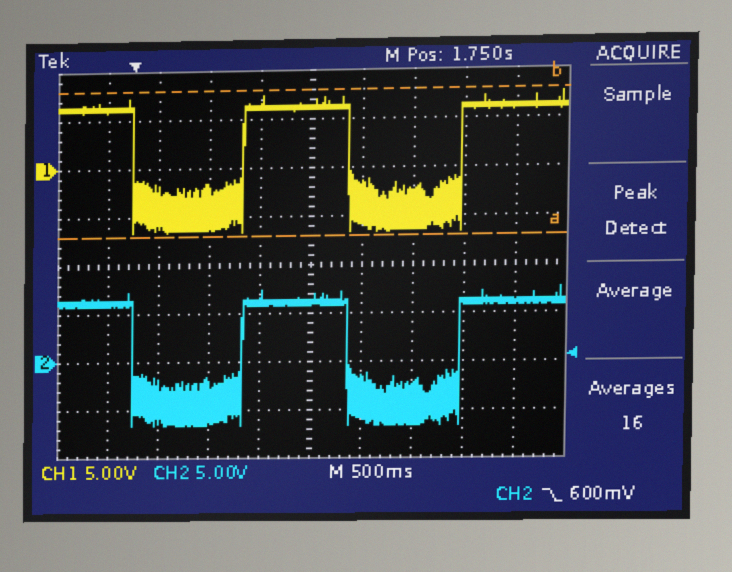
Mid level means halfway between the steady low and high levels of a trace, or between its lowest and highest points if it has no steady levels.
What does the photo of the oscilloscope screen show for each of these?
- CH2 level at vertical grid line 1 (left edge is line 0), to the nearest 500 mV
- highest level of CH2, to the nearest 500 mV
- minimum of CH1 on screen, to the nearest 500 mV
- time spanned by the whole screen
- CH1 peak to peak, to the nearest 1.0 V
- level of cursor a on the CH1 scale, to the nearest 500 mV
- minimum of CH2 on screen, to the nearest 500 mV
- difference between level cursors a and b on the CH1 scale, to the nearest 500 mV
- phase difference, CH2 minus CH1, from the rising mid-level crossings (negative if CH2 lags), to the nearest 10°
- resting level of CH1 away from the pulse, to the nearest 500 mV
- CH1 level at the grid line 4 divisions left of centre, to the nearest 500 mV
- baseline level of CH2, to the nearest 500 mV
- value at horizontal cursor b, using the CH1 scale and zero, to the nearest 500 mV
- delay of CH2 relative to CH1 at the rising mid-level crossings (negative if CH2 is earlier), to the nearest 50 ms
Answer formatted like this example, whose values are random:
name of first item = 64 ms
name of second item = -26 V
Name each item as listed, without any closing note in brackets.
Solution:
CH2 level at vertical grid line 1 (left edge is line 0), to the nearest 500 mV = 6.0 V
highest level of CH2, to the nearest 500 mV = 7.5 V
minimum of CH1 on screen, to the nearest 500 mV = -6.5 V
time spanned by the whole screen = 5 s
CH1 peak to peak, to the nearest 1.0 V = 14.0 V
level of cursor a on the CH1 scale, to the nearest 500 mV = -7.0 V
minimum of CH2 on screen, to the nearest 500 mV = -6.5 V
difference between level cursors a and b on the CH1 scale, to the nearest 500 mV = 15.0 V
phase difference, CH2 minus CH1, from the rising mid-level crossings (negative if CH2 lags), to the nearest 10° = 0°
resting level of CH1 away from the pulse, to the nearest 500 mV = 6.0 V
CH1 level at the grid line 4 divisions left of centre, to the nearest 500 mV = 6.0 V
baseline level of CH2, to the nearest 500 mV = 6.0 V
value at horizontal cursor b, using the CH1 scale and zero, to the nearest 500 mV = 8.0 V
delay of CH2 relative to CH1 at the rising mid-level crossings (negative if CH2 is earlier), to the nearest 50 ms = 0 ms
